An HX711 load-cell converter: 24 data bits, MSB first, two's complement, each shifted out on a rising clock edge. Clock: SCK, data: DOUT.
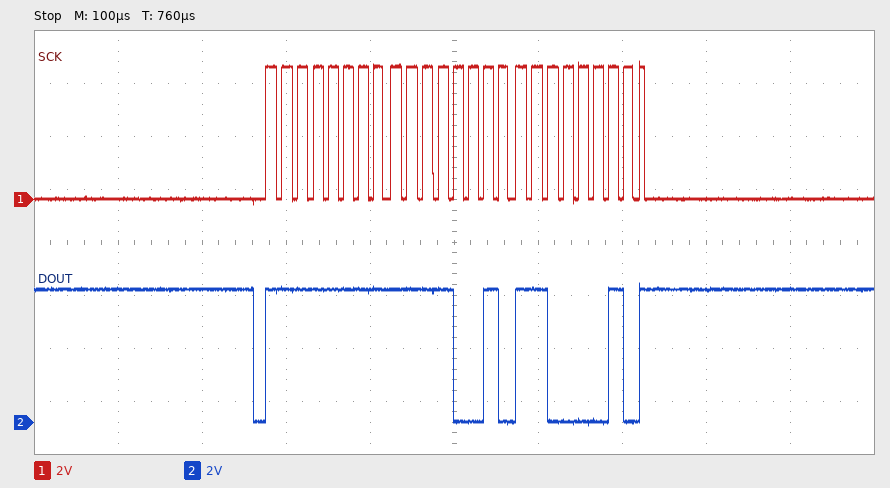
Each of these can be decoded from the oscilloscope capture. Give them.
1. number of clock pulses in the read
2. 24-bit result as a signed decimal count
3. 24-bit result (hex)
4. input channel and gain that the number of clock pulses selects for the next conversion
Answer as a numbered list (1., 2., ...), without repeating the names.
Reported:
1. 25
2. -3390
3. 0xFFF2C2
4. channel A, gain 128
